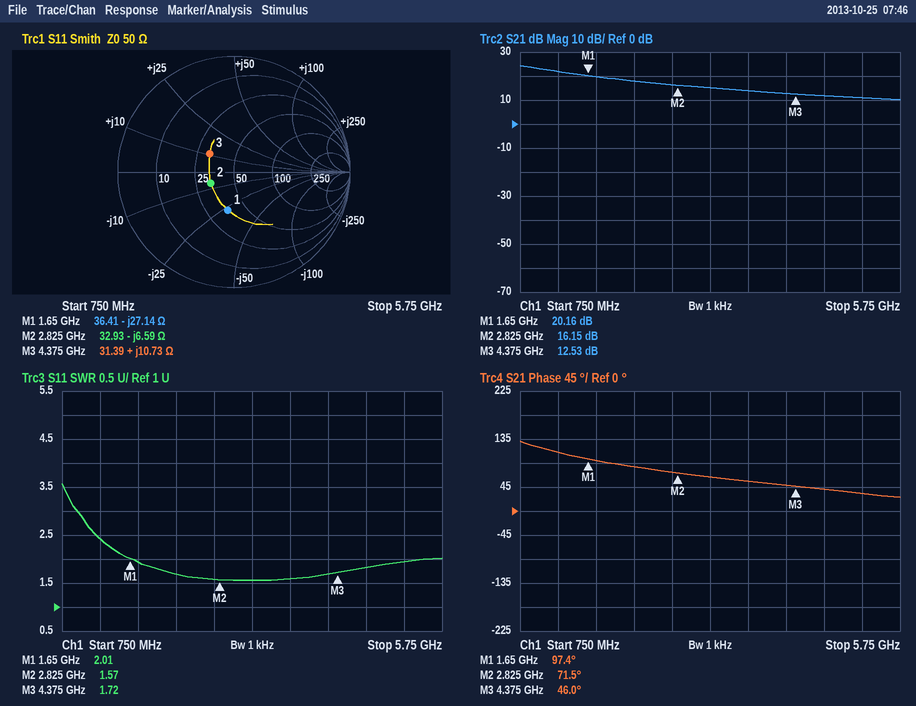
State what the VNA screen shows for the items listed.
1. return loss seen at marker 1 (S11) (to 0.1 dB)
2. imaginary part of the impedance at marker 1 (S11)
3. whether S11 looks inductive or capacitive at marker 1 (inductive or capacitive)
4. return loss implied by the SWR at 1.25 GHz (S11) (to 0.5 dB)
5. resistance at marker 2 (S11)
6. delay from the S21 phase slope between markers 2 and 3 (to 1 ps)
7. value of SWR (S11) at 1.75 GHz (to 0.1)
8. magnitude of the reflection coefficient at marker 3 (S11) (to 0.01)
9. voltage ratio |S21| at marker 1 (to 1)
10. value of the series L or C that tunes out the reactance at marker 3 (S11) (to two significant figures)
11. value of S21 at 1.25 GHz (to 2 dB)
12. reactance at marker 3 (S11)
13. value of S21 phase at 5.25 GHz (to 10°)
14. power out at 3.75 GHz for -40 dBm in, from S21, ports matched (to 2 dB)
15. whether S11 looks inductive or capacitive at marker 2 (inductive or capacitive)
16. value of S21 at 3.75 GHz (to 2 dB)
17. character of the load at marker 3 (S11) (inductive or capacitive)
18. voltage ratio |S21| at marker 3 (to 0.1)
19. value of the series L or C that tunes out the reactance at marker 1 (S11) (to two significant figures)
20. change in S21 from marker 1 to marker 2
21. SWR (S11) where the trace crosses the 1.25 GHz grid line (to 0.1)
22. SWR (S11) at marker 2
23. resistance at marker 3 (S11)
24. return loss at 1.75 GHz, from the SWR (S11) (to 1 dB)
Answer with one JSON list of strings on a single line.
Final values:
["9.5 dB", "-27.14 Ω", "capacitive", "7.5 dB", "32.93 Ω", "46 ps", "1.9", "0.26", "10", "3.4 pF", "22 dB", "+10.73 Ω", "30°", "-26 dBm", "capacitive", "14 dB", "inductive", "4.2", "2.6 nH", "-4.01 dB", "2.4", "1.57", "31.39 Ω", "10 dB"]
